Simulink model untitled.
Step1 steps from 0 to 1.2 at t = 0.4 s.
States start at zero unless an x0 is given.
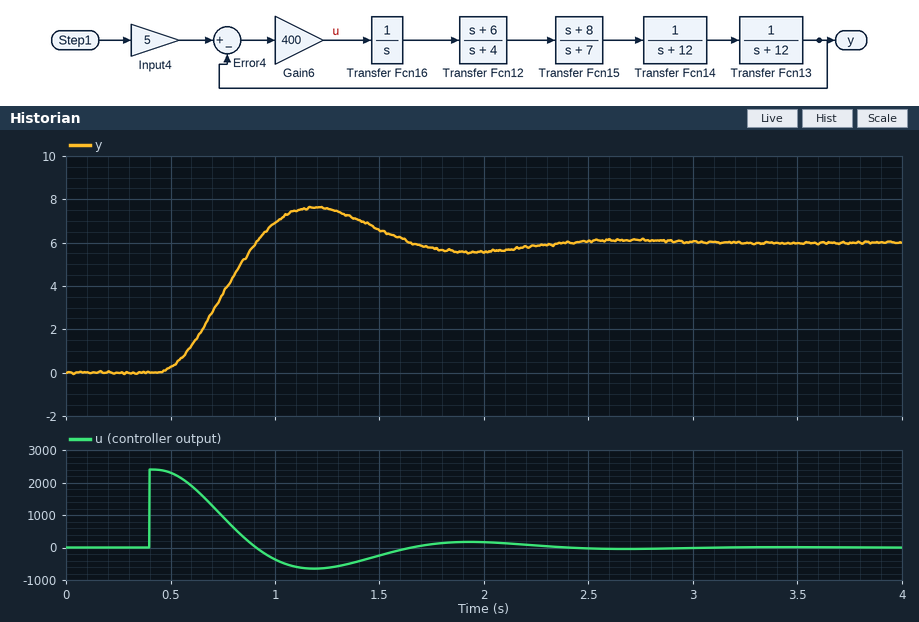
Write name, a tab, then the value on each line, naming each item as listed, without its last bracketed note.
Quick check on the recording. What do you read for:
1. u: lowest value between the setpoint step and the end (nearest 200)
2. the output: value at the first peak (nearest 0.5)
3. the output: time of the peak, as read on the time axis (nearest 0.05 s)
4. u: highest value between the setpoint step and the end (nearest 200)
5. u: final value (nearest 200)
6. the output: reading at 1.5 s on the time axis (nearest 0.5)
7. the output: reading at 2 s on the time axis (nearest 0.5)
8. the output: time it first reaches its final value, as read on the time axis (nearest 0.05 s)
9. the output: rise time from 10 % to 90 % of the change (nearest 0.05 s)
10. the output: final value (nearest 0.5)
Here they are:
u: lowest value between the setpoint step and the end	-600
the output: value at the first peak	7.5
the output: time of the peak, as read on the time axis	1.20 s
u: highest value between the setpoint step and the end	2400
u: final value	0
the output: reading at 1.5 s on the time axis	6.5
the output: reading at 2 s on the time axis	5.5
the output: time it first reaches its final value, as read on the time axis	0.90 s
the output: rise time from 10 % to 90 % of the change	0.30 s
the output: final value	6.0
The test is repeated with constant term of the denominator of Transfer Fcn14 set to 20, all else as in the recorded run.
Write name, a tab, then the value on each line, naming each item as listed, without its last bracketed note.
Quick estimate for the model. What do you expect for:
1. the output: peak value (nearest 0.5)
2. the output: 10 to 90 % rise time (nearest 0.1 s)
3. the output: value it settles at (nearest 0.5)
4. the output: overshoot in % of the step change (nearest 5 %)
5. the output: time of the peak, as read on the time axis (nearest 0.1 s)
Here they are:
the output: peak value	6.5
the output: 10 to 90 % rise time	0.5 s
the output: value it settles at	6.0
the output: overshoot in % of the step change	10 %
the output: time of the peak, as read on the time axis	1.5 s
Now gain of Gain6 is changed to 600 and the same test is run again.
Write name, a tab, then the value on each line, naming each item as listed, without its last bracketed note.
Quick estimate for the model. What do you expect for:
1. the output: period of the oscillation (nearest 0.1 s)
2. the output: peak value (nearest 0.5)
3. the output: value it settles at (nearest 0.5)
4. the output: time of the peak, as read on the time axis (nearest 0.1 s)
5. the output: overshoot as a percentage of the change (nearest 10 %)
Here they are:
the output: period of the oscillation	1.2 s
the output: peak value	8.5
the output: value it settles at	6.0
the output: time of the peak, as read on the time axis	1.0 s
the output: overshoot as a percentage of the change	40 %
